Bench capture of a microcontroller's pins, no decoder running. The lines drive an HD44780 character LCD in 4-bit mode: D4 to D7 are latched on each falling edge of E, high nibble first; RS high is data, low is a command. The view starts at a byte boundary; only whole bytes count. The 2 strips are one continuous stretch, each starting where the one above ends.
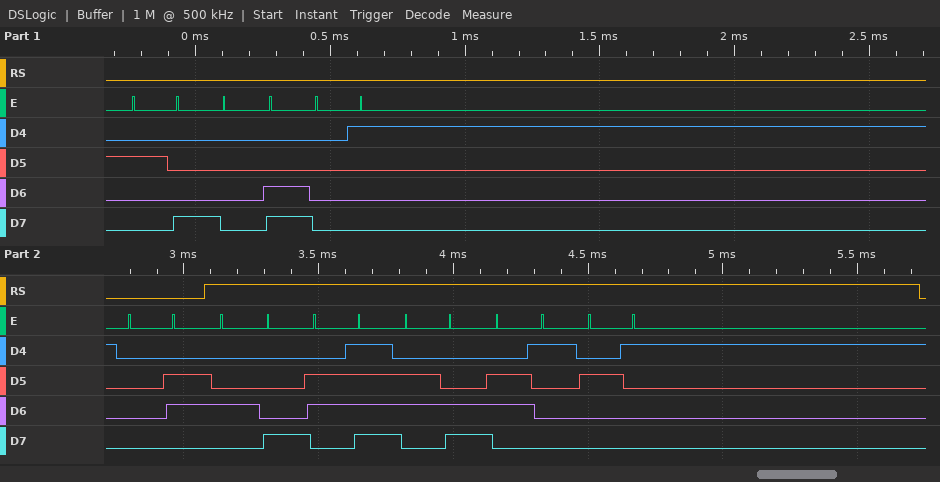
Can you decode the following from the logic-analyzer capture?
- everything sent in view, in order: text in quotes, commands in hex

0x28 0x0C 0x01 0x06 "Hola!"
